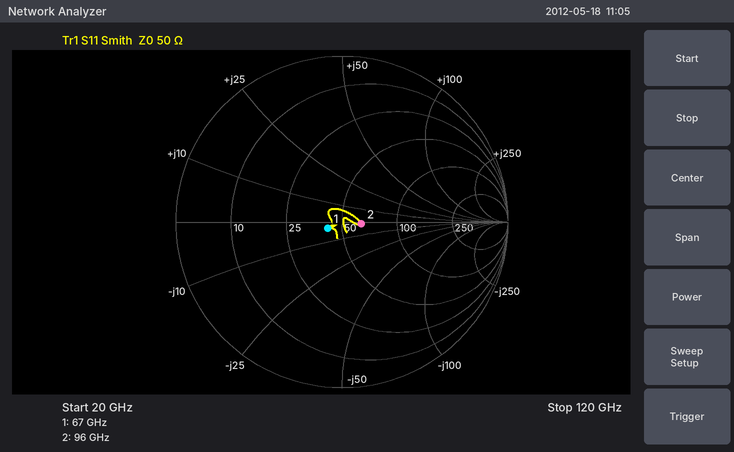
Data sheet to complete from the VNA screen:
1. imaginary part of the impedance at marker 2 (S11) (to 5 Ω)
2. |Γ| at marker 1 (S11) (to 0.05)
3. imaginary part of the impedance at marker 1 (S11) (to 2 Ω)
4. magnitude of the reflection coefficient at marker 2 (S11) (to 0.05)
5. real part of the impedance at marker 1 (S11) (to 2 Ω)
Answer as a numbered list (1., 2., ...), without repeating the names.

1. 0 Ω
2. 0.10
3. -4 Ω
4. 0.10
5. 42 Ω
